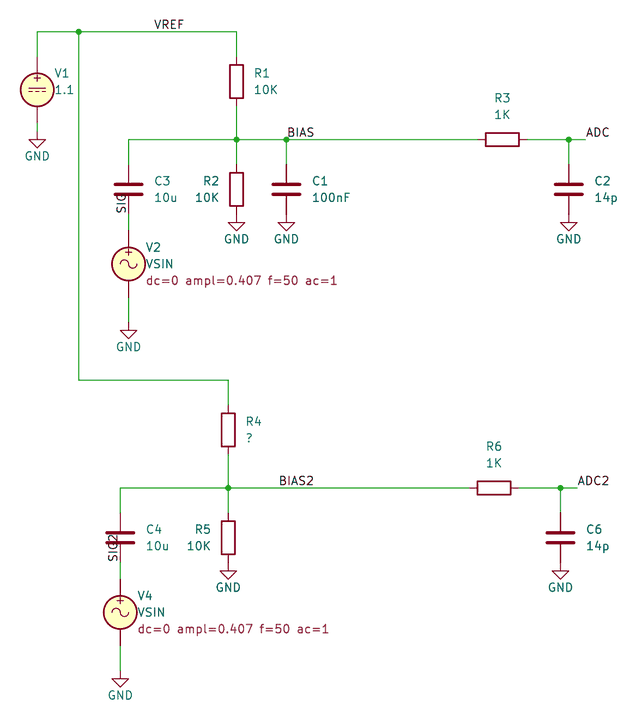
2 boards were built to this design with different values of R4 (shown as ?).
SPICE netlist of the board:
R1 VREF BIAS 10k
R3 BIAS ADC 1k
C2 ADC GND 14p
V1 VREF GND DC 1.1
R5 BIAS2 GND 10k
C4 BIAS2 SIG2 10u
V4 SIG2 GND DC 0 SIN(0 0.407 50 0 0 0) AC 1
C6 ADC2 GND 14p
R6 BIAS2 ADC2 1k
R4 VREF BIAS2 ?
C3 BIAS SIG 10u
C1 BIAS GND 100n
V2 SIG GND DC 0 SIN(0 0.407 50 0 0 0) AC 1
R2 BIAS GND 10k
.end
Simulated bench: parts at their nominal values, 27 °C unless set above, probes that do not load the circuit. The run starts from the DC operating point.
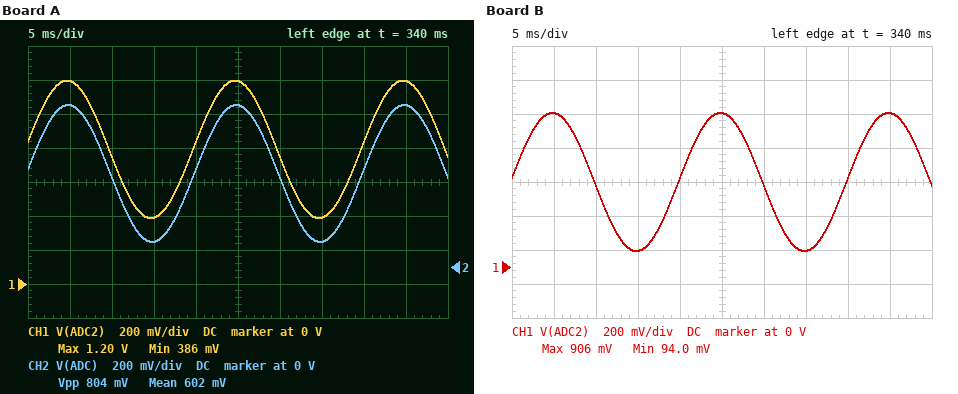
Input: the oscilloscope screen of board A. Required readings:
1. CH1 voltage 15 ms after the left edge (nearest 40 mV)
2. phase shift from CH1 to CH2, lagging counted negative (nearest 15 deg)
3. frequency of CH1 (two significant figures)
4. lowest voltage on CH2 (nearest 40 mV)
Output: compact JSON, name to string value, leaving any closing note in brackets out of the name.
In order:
{"CH1 voltage 15 ms after the left edge": "400 mV", "phase shift from CH1 to CH2, lagging counted negative": "0 deg", "frequency of CH1": "50 Hz", "lowest voltage on CH2": "160 mV"}
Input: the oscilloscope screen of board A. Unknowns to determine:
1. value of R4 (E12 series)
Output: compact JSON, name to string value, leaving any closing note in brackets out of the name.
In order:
{"value of R4": "3.9 kΩ"}
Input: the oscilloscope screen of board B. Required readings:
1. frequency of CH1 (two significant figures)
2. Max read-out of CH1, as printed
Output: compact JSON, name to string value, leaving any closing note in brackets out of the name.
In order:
{"frequency of CH1": "50 Hz", "Max read-out of CH1, as printed": "906 mV"}
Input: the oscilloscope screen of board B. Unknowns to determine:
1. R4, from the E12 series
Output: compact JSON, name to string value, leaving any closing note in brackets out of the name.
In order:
{"R4, from the E12 series": "12 kΩ"}
